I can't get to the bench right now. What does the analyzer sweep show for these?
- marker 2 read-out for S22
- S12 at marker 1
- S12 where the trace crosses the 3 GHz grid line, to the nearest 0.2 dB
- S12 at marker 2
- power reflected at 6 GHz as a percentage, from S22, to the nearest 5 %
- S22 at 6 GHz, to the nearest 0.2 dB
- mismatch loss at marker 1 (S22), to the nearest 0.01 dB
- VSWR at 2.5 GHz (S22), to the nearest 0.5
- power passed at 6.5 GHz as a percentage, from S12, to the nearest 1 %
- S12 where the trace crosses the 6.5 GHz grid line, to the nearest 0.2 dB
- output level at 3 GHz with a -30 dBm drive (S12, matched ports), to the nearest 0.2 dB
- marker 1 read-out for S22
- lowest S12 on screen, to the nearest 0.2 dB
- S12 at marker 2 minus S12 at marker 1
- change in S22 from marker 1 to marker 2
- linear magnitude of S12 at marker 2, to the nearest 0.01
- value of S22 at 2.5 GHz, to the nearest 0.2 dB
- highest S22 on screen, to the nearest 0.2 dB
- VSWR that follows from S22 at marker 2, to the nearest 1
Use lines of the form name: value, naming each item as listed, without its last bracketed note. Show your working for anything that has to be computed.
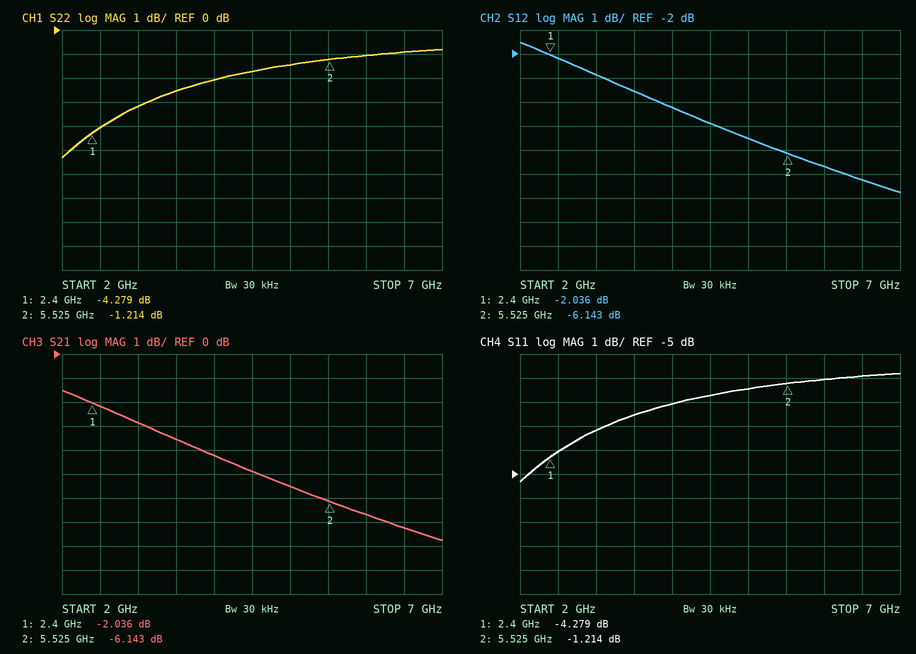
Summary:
marker 2 read-out for S22: -1.214 dB
S12 at marker 1: -2.036 dB
S12 where the trace crosses the 3 GHz grid line, to the nearest 0.2 dB: -2.8 dB
S12 at marker 2: -6.143 dB
power reflected at 6 GHz as a percentage, from S22, to the nearest 5 %: 10^(-1/10) ≈ 79.4 %, so 80 % to the nearest 5 %
S22 at 6 GHz, to the nearest 0.2 dB: -1.0 dB
mismatch loss at marker 1 (S22), to the nearest 0.01 dB: −10 log10(1 − 10^(-4.279/10)) ≈ 2.03 dB
VSWR at 2.5 GHz (S22), to the nearest 0.5: |Γ| = 10^(-4/20) = 0.6310; VSWR = (1 + 0.6310)/(1 − 0.6310) ≈ 4.42, so 4.5 to the nearest 0.5
power passed at 6.5 GHz as a percentage, from S12, to the nearest 1 %: 10^(-7.2/10) ≈ 19 %
S12 where the trace crosses the 6.5 GHz grid line, to the nearest 0.2 dB: -7.2 dB
output level at 3 GHz with a -30 dBm drive (S12, matched ports), to the nearest 0.2 dB: -30 dBm + (-2.8 dB) = -32.8 dBm
marker 1 read-out for S22: -4.279 dB
lowest S12 on screen, to the nearest 0.2 dB: -7.8 dB
S12 at marker 2 minus S12 at marker 1: -6.143 − (-2.036) = -4.107 dB
change in S22 from marker 1 to marker 2: -1.214 − (-4.279) = 3.065 dB
linear magnitude of S12 at marker 2, to the nearest 0.01: 10^(-6.143/20) ≈ 0.49
value of S22 at 2.5 GHz, to the nearest 0.2 dB: -4.0 dB
highest S22 on screen, to the nearest 0.2 dB: -0.8 dB
VSWR that follows from S22 at marker 2, to the nearest 1: (1 + 0.8696)/(1 − 0.8696) ≈ 14
